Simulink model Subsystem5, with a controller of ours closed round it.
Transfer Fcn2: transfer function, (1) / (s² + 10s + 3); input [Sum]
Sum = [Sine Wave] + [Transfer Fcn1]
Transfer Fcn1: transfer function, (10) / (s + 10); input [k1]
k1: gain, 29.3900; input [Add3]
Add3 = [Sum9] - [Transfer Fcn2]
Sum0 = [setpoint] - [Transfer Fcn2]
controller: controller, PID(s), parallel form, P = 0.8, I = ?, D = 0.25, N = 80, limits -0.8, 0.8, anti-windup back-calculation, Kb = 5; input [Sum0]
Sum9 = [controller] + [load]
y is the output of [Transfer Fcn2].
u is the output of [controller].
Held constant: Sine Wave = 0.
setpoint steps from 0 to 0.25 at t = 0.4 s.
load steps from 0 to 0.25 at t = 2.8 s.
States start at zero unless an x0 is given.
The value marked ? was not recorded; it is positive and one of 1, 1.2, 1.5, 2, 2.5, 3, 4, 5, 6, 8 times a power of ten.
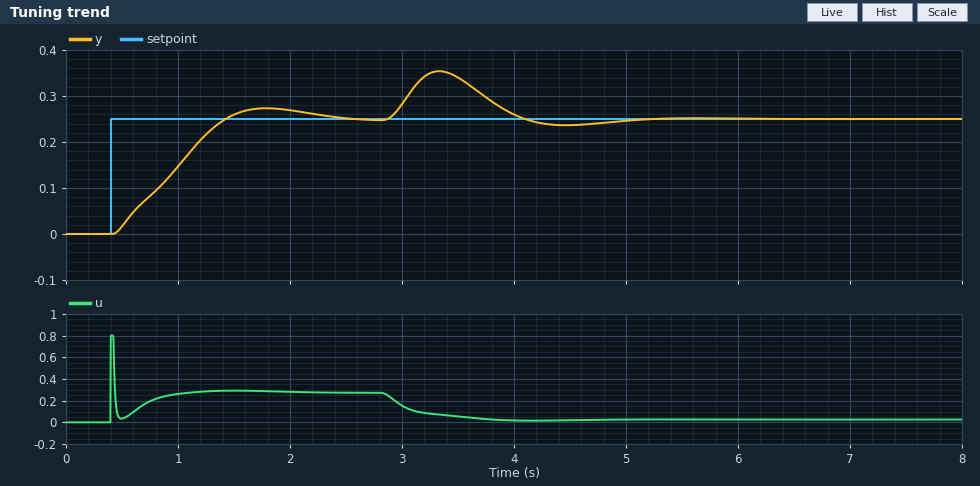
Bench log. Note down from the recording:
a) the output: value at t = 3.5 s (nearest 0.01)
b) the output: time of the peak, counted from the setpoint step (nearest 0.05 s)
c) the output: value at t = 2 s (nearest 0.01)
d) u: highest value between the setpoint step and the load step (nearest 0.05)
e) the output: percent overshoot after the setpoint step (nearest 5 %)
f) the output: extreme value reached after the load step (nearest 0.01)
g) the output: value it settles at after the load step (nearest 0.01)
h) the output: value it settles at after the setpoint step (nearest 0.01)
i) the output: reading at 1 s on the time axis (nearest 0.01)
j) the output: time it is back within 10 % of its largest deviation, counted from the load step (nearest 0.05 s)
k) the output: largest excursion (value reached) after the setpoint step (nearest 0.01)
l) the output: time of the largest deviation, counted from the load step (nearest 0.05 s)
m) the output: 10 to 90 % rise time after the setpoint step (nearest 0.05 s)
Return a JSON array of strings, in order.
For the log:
["0.34", "1.40 s", "0.27", "0.80", "10 %", "0.35", "0.25", "0.25", "0.15", "1.90 s", "0.27", "0.55 s", "0.75 s"]
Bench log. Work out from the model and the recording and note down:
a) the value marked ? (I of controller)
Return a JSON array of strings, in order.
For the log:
["4"]
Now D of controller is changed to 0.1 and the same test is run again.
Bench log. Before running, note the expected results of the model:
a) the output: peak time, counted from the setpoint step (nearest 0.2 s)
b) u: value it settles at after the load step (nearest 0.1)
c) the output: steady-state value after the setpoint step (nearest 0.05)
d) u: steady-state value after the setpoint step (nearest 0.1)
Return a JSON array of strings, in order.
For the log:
["0.8 s", "0.0", "0.25", "0.3"]
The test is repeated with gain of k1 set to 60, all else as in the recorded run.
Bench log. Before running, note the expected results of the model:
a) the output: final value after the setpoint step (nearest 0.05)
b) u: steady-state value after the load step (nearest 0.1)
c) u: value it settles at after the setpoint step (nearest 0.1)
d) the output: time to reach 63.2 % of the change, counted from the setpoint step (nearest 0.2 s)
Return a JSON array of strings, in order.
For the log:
["0.25", "0.0", "0.3", "0.6 s"]
